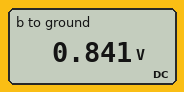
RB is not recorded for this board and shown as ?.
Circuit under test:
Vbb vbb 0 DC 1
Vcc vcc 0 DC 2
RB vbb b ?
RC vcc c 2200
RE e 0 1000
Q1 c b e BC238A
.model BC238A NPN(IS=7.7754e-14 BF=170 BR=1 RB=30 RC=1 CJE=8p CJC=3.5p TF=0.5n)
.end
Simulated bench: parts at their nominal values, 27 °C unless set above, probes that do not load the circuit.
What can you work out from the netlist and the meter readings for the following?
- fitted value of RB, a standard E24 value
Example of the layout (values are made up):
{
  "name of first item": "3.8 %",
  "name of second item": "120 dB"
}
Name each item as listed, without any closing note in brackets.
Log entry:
{
  "fitted value of RB, a standard E24 value": "100 kΩ"
}
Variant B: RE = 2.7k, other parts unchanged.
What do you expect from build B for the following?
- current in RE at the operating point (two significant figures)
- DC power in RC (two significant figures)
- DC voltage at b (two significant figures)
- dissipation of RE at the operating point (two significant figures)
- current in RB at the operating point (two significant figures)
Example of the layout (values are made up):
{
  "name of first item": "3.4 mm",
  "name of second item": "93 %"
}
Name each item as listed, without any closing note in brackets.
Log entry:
{
  "current in RE at the operating point": "140 µA",
  "DC power in RC": "41 µW",
  "DC voltage at b": "920 mV",
  "dissipation of RE at the operating point": "51 µW",
  "current in RB at the operating point": "800 nA"
}
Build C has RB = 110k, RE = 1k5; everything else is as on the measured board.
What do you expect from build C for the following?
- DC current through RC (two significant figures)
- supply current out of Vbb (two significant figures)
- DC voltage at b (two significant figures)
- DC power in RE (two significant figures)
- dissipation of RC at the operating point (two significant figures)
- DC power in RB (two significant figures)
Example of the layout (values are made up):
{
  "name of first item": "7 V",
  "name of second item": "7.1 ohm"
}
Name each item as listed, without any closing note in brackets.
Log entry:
{
  "DC current through RC": "200 µA",
  "supply current out of Vbb": "1.2 µA",
  "DC voltage at b": "870 mV",
  "DC power in RE": "63 µW",
  "dissipation of RC at the operating point": "91 µW",
  "DC power in RB": "160 nW"
}
